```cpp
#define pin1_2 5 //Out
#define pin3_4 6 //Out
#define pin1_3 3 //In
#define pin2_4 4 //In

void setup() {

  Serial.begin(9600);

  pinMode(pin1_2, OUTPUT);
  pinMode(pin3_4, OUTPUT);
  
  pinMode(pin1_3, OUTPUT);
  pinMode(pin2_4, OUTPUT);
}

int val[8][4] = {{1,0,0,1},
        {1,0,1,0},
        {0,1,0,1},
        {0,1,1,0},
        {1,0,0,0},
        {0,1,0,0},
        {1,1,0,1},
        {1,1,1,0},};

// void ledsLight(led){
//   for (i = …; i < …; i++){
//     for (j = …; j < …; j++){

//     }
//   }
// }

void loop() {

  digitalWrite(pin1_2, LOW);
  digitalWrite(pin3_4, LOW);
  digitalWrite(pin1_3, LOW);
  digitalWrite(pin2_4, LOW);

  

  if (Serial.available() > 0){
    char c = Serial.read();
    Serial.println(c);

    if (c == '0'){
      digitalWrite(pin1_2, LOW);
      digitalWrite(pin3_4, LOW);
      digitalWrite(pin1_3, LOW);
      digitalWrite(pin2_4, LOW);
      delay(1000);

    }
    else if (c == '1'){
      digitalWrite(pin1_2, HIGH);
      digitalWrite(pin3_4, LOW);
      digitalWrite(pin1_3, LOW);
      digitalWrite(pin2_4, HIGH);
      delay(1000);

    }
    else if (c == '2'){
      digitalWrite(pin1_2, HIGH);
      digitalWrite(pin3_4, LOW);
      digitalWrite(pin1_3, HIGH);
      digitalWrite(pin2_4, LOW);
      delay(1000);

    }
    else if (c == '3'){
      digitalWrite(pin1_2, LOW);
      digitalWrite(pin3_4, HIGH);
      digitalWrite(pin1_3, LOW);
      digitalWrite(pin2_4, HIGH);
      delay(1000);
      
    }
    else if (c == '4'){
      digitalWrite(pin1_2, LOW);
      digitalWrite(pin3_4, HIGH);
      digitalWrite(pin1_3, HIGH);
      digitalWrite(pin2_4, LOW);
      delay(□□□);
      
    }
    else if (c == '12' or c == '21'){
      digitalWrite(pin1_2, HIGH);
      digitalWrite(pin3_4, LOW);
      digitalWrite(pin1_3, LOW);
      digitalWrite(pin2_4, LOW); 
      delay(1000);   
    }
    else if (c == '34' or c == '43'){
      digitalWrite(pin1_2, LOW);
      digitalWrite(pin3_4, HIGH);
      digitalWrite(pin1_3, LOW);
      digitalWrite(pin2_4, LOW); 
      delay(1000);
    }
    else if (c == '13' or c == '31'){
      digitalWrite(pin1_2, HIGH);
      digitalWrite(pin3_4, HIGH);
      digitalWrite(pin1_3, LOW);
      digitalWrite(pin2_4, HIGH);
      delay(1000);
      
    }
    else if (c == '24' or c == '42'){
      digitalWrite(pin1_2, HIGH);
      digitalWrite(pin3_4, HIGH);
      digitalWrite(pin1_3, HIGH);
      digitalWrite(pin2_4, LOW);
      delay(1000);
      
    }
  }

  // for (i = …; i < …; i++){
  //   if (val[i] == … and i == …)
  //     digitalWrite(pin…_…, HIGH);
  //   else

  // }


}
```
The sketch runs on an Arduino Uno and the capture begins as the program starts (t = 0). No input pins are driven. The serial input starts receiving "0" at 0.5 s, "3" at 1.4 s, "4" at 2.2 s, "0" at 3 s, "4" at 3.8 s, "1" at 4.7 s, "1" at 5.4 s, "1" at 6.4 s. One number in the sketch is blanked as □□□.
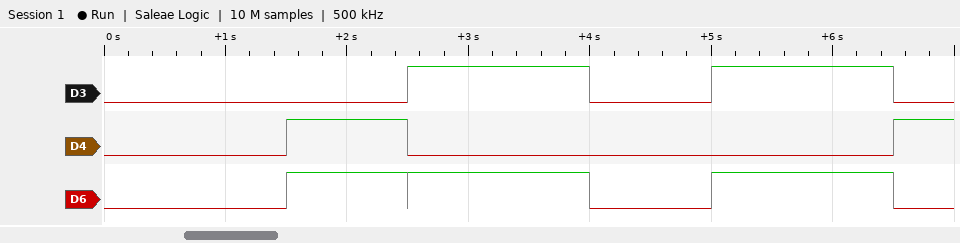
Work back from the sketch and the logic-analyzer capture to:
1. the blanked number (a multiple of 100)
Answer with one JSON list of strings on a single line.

["1500"]
